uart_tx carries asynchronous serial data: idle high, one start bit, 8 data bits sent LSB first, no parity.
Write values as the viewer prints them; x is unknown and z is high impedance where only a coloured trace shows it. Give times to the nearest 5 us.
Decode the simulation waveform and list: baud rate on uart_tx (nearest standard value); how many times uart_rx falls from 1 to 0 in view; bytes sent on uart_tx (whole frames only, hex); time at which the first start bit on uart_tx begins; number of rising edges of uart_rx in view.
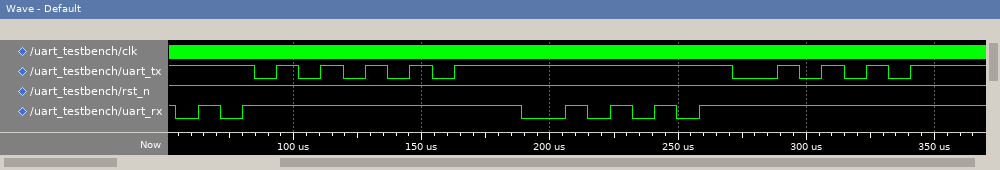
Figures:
115200 baud
6
55, AA
85 us
6
